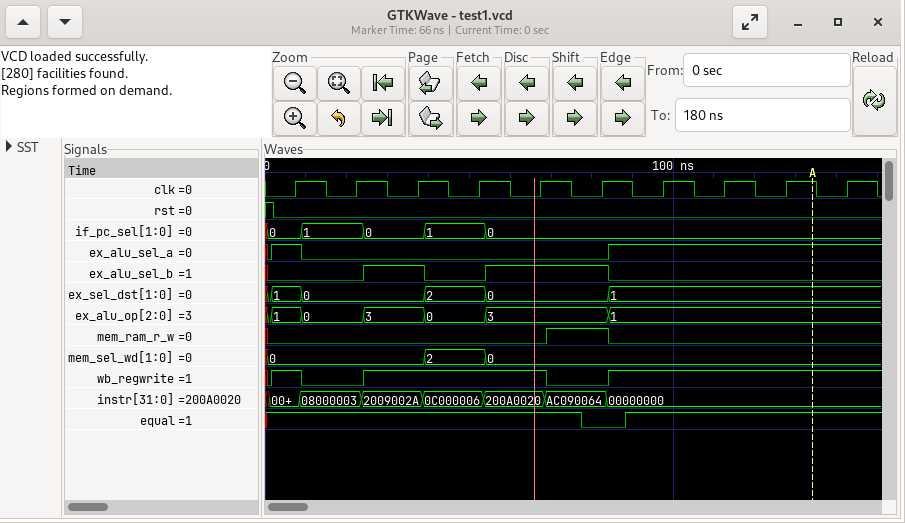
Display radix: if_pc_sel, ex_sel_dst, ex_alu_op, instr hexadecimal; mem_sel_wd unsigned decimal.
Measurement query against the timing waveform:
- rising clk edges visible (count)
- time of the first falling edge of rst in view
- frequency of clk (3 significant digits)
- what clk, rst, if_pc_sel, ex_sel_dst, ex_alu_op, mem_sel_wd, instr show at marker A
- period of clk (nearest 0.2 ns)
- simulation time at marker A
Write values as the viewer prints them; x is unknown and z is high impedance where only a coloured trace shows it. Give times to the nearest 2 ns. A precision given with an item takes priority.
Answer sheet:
10
2 ns
66.7 MHz
clk=1, rst=0, if_pc_sel=0, ex_sel_dst=1, ex_alu_op=1, mem_sel_wd=0, instr=00000000
15 ns
134 ns
